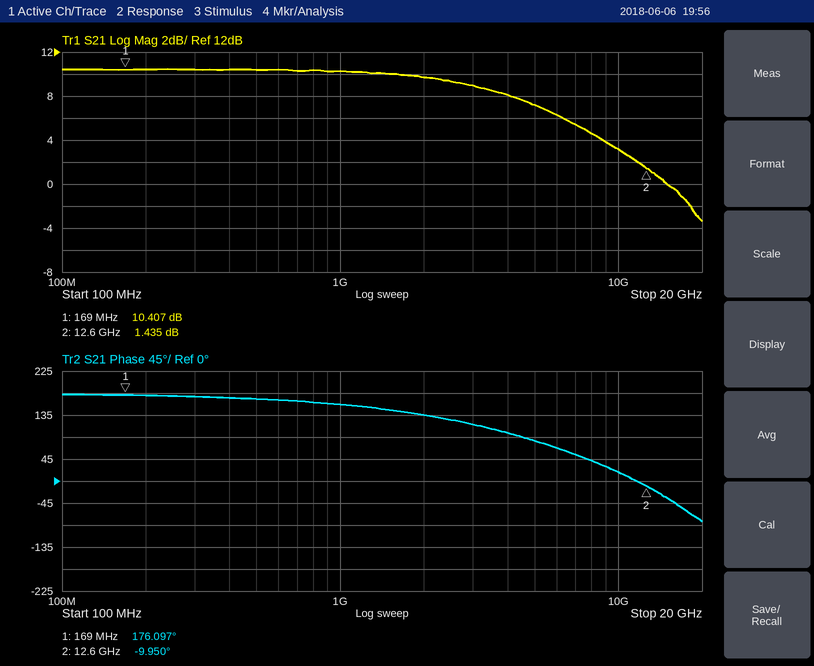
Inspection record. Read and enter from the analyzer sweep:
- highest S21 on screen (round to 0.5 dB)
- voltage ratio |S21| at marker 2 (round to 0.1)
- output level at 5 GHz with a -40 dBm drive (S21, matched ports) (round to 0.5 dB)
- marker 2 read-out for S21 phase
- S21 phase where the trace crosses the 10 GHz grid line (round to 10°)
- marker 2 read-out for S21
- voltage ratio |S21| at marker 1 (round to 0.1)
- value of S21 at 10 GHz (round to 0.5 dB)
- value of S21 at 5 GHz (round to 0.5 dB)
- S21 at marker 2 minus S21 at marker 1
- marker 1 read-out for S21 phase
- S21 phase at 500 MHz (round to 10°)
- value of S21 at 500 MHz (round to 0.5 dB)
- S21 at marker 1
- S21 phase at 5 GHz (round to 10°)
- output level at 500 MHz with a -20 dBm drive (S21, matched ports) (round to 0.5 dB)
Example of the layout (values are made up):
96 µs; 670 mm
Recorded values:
10.5 dB; 1.2; -33.0 dBm; -9.950°; 20°; 1.435 dB; 3.3; 3.0 dB; 7.0 dB; -8.972 dB; 176.097°; 170°; 10.5 dB; 10.407 dB; 80°; -9.5 dBm
